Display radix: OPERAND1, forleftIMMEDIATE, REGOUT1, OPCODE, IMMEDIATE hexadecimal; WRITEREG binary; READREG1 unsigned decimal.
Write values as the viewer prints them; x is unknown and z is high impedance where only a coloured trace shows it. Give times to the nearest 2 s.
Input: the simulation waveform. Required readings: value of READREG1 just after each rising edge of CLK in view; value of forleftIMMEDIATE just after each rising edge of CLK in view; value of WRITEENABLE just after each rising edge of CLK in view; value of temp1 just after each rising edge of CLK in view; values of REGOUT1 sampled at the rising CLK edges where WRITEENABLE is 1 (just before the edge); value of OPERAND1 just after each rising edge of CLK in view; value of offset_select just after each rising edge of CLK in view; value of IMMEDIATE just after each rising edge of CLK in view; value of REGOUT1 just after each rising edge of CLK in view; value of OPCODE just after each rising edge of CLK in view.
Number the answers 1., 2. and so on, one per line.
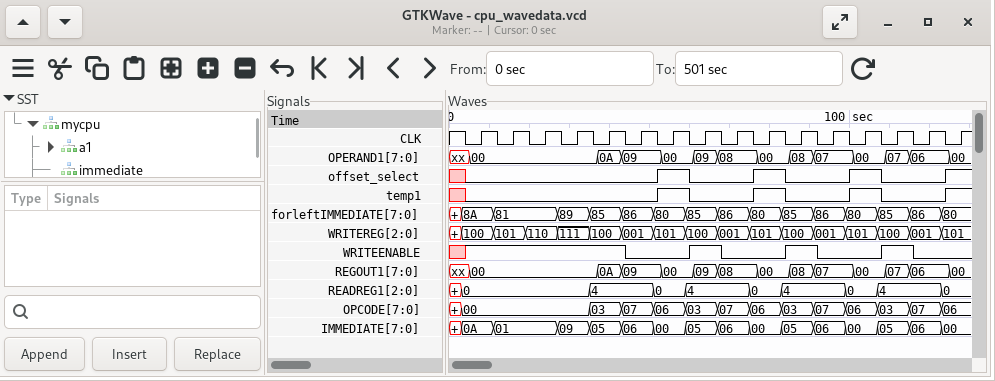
1. 0, 0, 0, 0, 4, 4, 0, 4, 4, 0, 4, 4, 0, 4, 4, 0
2. 8A, 81, 81, 89, 85, 86, 80, 85, 86, 80, 85, 86, 80, 85, 86, 80
3. 1 1 1 1 1 0 0 1 0 0 1 0 0 1 0 0
4. 0 0 0 0 0 0 1 0 0 1 0 0 1 0 0 1
5. 00, 00, 00, 00, 0A, 09, 08, 07
6. 00, 00, 00, 00, 0A, 09, 00, 09, 08, 00, 08, 07, 00, 07, 06, 00
7. 0 0 0 0 0 0 1 0 0 1 0 0 1 0 0 1
8. 0A, 01, 01, 09, 05, 06, 00, 05, 06, 00, 05, 06, 00, 05, 06, 00
9. 00, 00, 00, 00, 0A, 09, 00, 09, 08, 00, 08, 07, 00, 07, 06, 00
10. 00, 00, 00, 00, 03, 07, 06, 03, 07, 06, 03, 07, 06, 03, 07, 06
